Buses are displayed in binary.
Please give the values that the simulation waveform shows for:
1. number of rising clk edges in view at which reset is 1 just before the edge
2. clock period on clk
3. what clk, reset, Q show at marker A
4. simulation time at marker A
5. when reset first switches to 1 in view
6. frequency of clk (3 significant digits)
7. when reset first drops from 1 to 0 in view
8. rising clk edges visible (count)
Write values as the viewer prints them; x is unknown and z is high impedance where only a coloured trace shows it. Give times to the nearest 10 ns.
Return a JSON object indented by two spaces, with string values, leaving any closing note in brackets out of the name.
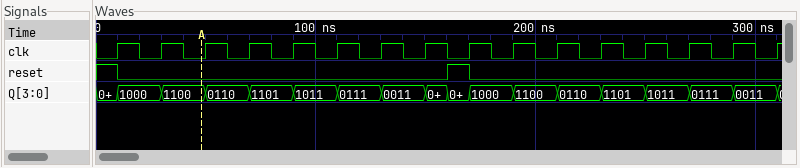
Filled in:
{
  "number of rising clk edges in view at which reset is 1 just before the edge": "2",
  "clock period on clk": "20 ns",
  "what clk, reset, Q show at marker A": "clk=0, reset=0, Q=1100",
  "simulation time at marker A": "50 ns",
  "when reset first switches to 1 in view": "160 ns",
  "frequency of clk": "50.0 MHz",
  "when reset first drops from 1 to 0 in view": "10 ns",
  "rising clk edges visible": "16"
}
